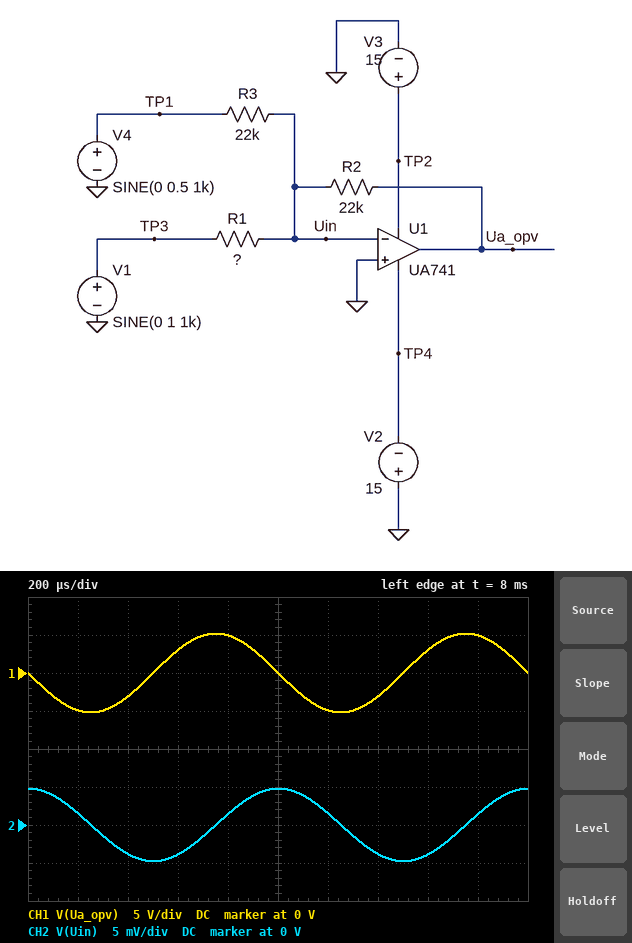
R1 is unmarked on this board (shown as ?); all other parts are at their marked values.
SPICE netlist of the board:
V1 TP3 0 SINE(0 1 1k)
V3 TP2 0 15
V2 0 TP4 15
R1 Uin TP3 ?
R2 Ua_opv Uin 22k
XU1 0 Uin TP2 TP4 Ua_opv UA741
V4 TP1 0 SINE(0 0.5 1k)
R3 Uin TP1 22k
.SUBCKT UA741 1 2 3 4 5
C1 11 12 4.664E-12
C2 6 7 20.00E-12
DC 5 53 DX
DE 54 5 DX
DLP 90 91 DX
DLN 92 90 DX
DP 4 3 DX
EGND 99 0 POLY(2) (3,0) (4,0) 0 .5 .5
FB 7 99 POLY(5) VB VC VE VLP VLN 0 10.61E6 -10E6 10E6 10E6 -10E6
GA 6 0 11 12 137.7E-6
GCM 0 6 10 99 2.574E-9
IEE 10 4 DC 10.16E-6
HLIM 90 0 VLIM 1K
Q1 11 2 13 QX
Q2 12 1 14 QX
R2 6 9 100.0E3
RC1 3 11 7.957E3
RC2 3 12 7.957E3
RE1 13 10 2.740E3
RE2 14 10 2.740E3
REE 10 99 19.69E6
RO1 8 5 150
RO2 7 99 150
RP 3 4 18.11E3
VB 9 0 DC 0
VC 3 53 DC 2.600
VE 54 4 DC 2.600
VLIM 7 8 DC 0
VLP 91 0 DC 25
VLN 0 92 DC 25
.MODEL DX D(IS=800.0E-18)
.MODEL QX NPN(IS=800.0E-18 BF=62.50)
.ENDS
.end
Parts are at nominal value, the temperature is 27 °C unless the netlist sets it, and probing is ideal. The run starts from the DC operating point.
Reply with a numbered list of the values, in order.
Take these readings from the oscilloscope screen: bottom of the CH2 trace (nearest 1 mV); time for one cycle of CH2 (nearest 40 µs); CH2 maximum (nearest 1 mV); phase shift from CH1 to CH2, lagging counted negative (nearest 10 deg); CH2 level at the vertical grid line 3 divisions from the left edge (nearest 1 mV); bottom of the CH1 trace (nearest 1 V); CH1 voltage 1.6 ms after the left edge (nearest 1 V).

1. -5 mV
2. 1.00 ms
3. 5 mV
4. -90 deg
5. -4 mV
6. -5 V
7. 3 V
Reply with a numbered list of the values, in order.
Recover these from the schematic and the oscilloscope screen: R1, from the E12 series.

1. 4.7 kΩ
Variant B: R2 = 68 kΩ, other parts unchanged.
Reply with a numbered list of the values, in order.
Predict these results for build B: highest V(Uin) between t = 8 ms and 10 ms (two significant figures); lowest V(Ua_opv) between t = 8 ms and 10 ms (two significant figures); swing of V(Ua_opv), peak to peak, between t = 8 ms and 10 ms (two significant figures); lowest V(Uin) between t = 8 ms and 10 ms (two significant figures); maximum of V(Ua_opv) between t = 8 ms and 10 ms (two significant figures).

1. 160 mV
2. -13 V
3. 26 V
4. -160 mV
5. 13 V
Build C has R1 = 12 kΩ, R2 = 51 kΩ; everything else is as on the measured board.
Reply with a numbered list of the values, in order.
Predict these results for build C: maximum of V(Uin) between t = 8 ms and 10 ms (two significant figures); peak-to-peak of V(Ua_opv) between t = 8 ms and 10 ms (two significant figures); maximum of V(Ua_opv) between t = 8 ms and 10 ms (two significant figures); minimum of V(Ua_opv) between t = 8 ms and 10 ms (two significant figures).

1. 5.0 mV
2. 11 V
3. 5.4 V
4. -5.4 V
